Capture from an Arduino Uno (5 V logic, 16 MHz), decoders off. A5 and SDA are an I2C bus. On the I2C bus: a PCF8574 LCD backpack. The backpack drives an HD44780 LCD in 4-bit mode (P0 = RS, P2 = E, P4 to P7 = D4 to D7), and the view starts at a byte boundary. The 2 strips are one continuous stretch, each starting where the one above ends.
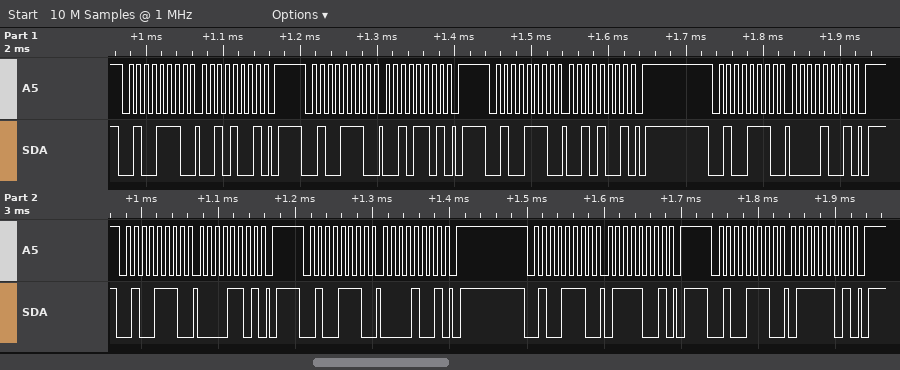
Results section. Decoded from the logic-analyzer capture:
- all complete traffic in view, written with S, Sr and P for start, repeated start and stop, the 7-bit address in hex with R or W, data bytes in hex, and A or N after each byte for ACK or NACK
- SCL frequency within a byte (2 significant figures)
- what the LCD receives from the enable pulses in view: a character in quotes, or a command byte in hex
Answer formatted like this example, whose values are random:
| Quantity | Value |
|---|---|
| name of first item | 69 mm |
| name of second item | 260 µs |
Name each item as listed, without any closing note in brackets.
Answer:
| Quantity | Value |
|---|---|
| all complete traffic in view, written with S, Sr and P for start, repeated start and stop, the 7-bit address in hex with R or W, data bytes in hex, and A or N after each byte for ACK or NACK | S 27W A 29 A P S 27W A 2D A P S 27W A 29 A P S 27W A 09 A P S 27W A 0D A P S 27W A 09 A P S 27W A 79 A P S 27W A 7D A P |
| SCL frequency within a byte | 100 kHz |
| what the LCD receives from the enable pulses in view: a character in quotes, or a command byte in hex | ' ' |
